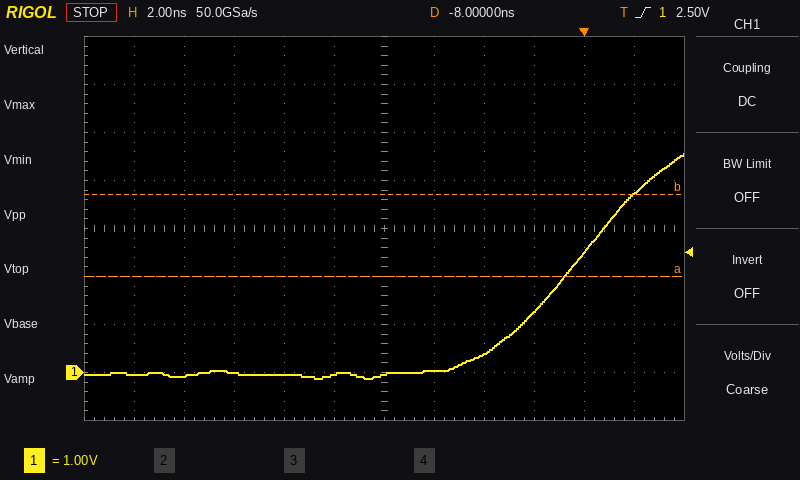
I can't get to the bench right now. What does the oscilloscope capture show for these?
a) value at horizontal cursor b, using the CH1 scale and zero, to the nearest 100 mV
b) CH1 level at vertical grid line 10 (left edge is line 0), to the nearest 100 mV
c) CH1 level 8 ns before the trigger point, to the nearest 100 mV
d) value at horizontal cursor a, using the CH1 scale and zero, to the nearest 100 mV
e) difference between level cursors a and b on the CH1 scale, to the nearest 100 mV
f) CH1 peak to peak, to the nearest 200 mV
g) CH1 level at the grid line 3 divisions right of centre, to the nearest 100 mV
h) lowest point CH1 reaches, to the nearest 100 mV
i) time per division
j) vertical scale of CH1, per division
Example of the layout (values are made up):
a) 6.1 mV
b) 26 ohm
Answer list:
a) 3.7 V
b) 2.5 V
c) 0.0 V
d) 2.0 V
e) 1.7 V
f) 4.6 V
g) 1.3 V
h) -100 mV
i) 2 ns
j) 1 V
